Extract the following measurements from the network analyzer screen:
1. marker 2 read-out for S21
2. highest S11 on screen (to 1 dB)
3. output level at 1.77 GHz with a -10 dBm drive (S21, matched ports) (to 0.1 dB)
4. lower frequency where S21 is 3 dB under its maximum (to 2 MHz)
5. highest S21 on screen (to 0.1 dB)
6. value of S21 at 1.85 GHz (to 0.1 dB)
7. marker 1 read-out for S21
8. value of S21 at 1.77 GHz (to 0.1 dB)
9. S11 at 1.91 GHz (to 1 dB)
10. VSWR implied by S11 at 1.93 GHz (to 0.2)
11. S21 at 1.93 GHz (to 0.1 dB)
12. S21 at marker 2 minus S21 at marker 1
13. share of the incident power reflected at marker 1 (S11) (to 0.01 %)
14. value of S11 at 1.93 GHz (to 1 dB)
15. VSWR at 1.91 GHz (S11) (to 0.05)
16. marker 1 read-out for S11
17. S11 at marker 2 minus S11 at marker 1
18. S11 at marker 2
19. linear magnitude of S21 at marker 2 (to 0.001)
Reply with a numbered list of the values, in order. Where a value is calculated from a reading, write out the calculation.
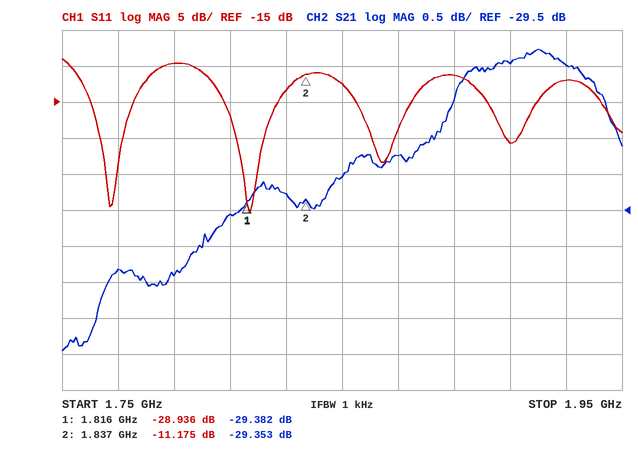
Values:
1. -29.353 dB
2. -9 dB
3. -10 dBm + (-30.3 dB) = -40.3 dBm
4. 1.794 GHz
5. -27.3 dB
6. -29.0 dB
7. -29.382 dB
8. -30.3 dB
9. -21 dB
10. |Γ| = 10^(-12/20) = 0.2512; VSWR = (1 + 0.2512)/(1 − 0.2512) ≈ 1.67, so 1.6 to the nearest 0.2
11. -27.5 dB
12. -29.353 − (-29.382) = 0.029 dB
13. 10^(-28.936/10) ≈ 0.13 %
14. -12 dB
15. |Γ| = 10^(-21/20) = 0.0891; VSWR = (1 + 0.0891)/(1 − 0.0891) ≈ 1.20
16. -28.936 dB
17. -11.175 − (-28.936) = 17.761 dB
18. -11.175 dB
19. 10^(-29.353/20) ≈ 0.034
